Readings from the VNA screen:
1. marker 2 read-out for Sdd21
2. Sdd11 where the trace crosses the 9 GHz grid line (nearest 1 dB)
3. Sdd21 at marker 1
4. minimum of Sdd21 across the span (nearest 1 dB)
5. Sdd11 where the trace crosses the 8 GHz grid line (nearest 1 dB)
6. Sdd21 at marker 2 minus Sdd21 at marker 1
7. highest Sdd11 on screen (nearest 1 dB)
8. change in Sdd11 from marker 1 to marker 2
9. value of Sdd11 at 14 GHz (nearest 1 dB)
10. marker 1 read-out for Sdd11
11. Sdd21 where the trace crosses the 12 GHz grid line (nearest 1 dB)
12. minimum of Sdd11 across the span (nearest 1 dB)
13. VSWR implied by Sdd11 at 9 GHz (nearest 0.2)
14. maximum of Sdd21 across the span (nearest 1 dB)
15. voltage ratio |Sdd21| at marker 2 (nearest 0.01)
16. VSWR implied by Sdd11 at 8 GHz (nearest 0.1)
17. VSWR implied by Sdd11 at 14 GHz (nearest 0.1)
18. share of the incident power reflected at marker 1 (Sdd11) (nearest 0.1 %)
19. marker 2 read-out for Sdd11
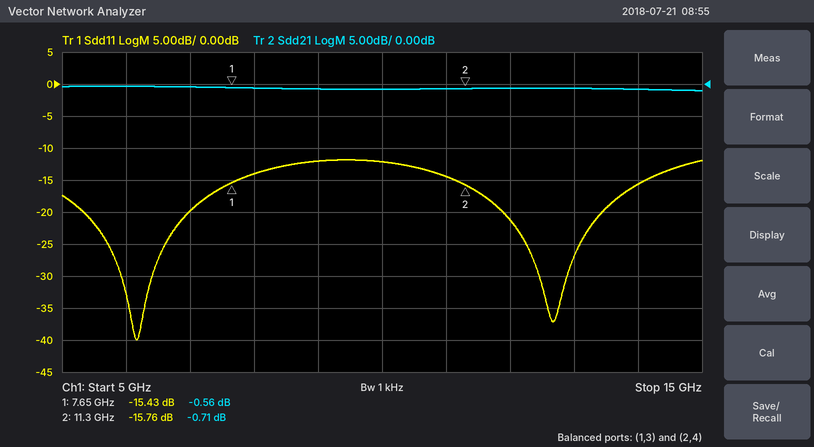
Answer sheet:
-0.71 dB
-12 dB
-0.56 dB
-1 dB
-14 dB
-0.15 dB
-12 dB
-0.33 dB
-16 dB
-15.43 dB
-1 dB
-40 dB
1.6
0 dB
0.92
1.5
1.4
2.9 %
-15.76 dB
